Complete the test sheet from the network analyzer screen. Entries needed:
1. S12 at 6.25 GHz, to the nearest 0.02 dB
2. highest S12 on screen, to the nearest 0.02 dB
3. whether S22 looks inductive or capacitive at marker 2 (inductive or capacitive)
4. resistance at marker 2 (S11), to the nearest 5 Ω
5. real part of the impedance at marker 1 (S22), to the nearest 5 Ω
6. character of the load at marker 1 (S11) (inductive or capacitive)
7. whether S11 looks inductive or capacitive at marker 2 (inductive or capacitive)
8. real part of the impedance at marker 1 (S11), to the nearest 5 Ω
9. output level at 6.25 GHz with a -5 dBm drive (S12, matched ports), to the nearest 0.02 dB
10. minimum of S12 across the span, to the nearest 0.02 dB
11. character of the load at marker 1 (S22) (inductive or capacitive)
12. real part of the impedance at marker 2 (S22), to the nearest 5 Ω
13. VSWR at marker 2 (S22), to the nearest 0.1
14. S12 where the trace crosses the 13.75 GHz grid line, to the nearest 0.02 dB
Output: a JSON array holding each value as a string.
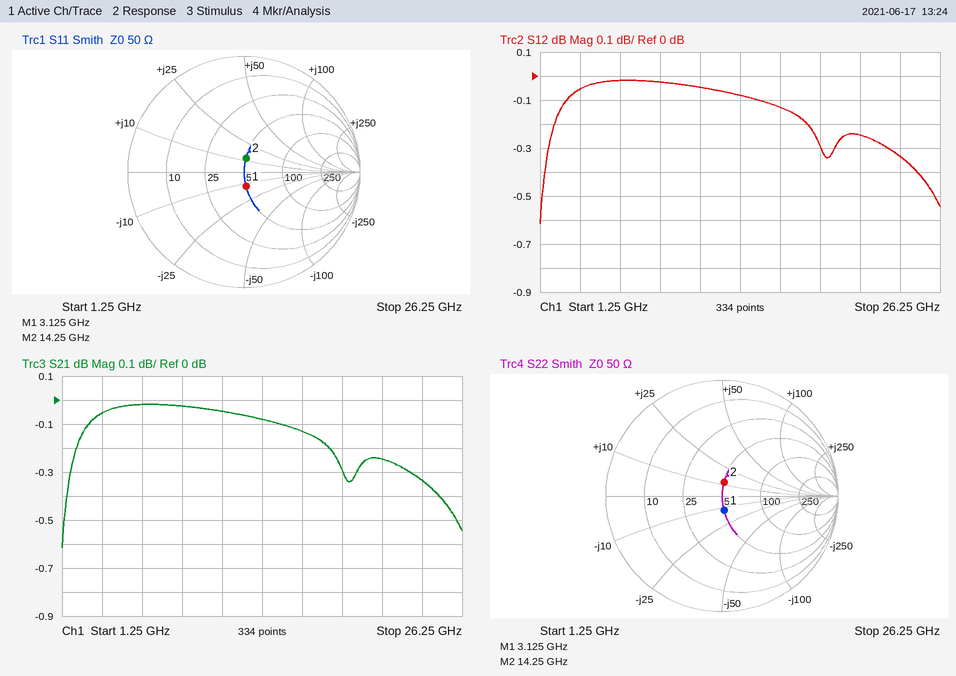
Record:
["-0.02 dB", "-0.02 dB", "inductive", "50 Ω", "50 Ω", "capacitive", "inductive", "50 Ω", "-5.02 dBm", "-0.62 dB", "capacitive", "50 Ω", "1.3", "-0.08 dB"]
